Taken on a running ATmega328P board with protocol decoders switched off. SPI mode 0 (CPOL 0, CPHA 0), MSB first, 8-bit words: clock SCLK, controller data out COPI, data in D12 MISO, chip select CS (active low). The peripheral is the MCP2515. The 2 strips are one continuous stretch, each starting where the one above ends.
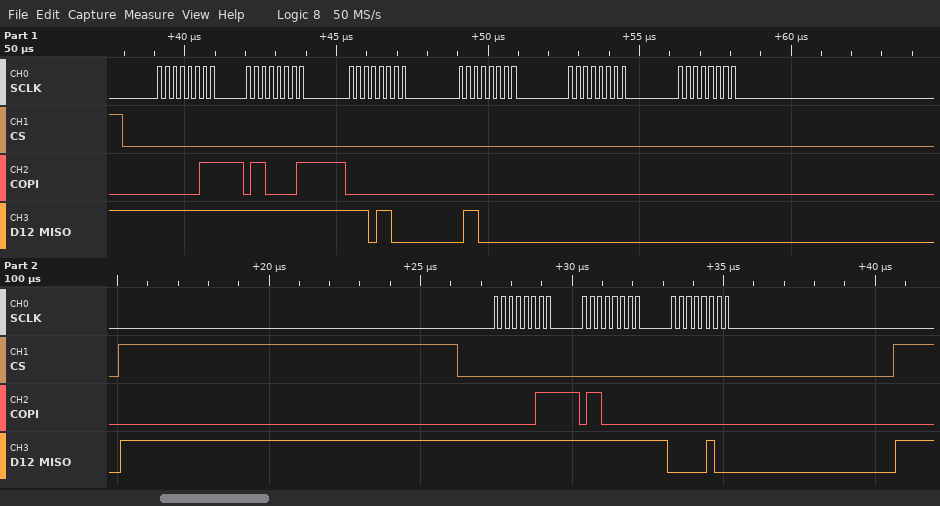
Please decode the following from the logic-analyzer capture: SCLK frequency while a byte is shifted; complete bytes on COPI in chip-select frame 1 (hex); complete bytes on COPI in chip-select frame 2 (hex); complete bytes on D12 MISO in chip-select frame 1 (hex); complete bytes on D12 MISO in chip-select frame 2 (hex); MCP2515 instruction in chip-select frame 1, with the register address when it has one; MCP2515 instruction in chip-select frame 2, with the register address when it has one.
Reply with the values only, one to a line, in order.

4 MHz
03 61 00 00 00 00
03 60 00
FF FF EC 60 00 00
FF FF 04
READ 0x61
READ 0x60
